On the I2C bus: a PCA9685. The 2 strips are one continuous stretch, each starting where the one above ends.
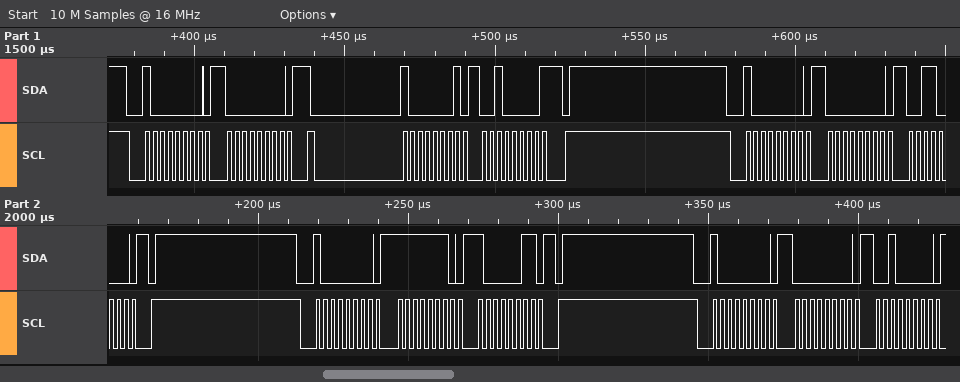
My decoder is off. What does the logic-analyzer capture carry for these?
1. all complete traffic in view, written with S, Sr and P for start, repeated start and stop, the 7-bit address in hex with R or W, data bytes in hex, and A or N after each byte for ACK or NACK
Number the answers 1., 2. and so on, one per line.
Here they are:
1. S 40W A 00 A Sr 40R A 20 N P S 40W A 00 A 30 A P S 40W A FE A 83 A P S 40W A 00 A 20 A
